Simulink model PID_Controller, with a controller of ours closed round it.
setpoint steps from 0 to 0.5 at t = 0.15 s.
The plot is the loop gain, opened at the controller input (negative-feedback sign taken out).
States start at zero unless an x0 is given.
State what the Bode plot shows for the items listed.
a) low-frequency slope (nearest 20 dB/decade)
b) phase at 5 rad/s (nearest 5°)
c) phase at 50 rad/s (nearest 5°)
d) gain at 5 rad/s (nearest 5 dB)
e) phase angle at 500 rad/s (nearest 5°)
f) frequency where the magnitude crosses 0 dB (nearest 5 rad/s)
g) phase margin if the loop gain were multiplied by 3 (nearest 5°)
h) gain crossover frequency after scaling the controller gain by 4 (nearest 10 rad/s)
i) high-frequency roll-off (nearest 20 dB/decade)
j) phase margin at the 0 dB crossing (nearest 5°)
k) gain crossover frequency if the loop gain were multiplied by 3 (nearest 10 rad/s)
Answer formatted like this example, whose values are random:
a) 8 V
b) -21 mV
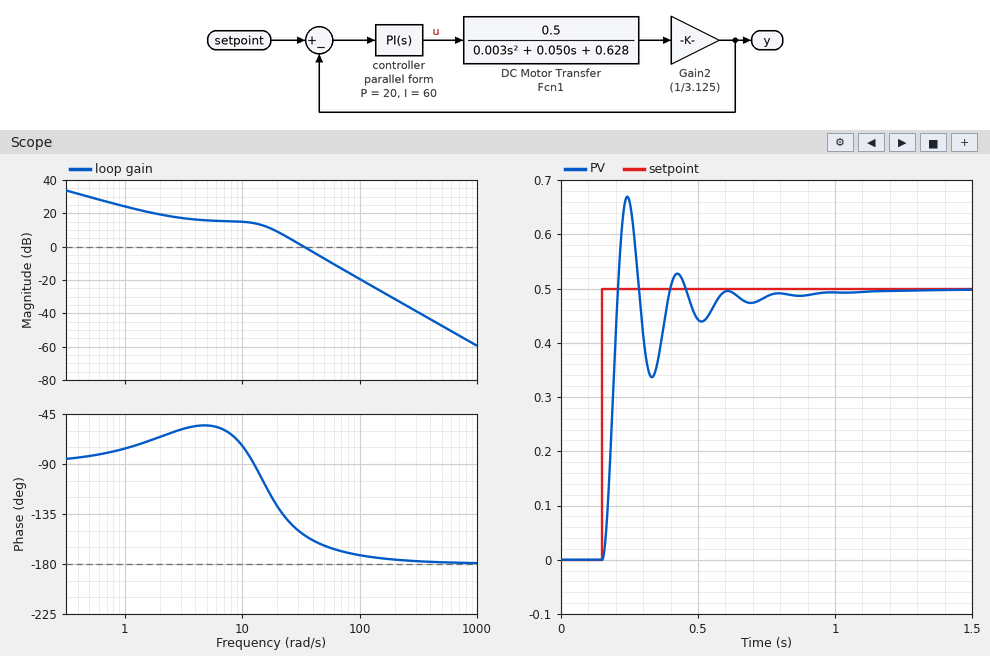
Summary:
a) -20 dB/decade
b) -55°
c) -165°
d) 15 dB
e) -180°
f) 35 rad/s
g) 15°
h) 70 rad/s
i) -40 dB/decade
j) 25°
k) 60 rad/s
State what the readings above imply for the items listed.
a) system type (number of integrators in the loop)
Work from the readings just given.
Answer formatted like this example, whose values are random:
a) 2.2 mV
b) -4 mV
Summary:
a) 1
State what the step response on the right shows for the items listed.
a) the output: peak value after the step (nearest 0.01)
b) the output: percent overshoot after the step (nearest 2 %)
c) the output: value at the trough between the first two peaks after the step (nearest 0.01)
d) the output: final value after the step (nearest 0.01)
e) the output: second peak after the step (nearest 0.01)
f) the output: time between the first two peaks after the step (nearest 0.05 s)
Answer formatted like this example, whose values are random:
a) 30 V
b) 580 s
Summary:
a) 0.67
b) 34 %
c) 0.34
d) 0.50
e) 0.53
f) 0.20 s
